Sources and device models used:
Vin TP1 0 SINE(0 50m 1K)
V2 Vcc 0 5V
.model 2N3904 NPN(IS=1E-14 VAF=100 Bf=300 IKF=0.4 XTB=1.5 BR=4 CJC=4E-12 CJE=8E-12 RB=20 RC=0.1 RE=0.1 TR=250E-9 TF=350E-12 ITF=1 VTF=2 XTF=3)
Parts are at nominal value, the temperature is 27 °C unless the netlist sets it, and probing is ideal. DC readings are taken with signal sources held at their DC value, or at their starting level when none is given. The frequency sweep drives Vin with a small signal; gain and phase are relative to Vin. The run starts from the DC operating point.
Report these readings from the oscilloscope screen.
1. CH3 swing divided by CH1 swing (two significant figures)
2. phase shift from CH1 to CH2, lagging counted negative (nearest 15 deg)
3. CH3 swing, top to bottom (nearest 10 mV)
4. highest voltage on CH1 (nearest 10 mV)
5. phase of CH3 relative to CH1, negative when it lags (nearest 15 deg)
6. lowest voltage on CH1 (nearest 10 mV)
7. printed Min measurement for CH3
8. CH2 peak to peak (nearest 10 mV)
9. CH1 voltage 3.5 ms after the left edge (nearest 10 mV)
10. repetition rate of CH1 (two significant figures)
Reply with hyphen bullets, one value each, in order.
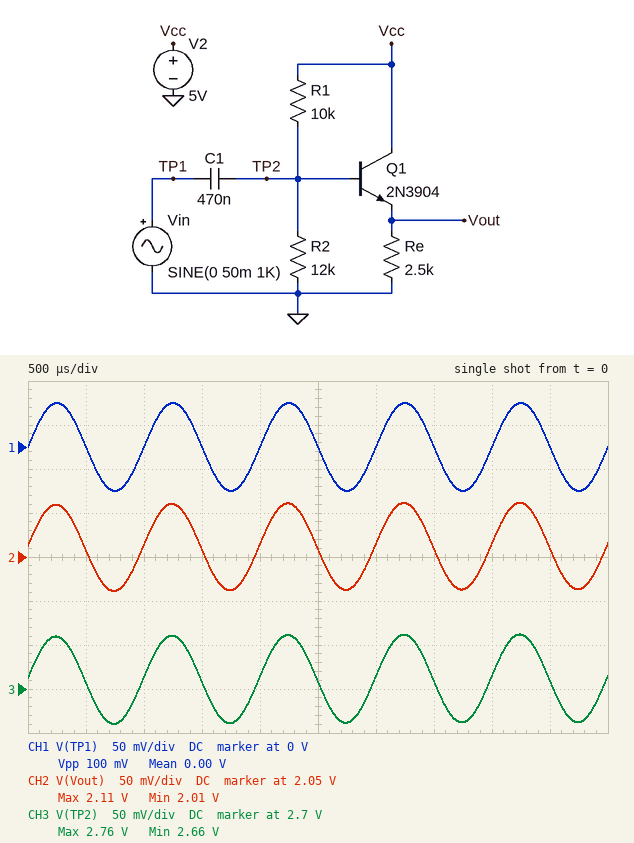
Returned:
- 1.0
- 0 deg
- 100 mV
- 50 mV
- 0 deg
- -50 mV
- 2.66 V
- 100 mV
- 0 V
- 1.0 kHz
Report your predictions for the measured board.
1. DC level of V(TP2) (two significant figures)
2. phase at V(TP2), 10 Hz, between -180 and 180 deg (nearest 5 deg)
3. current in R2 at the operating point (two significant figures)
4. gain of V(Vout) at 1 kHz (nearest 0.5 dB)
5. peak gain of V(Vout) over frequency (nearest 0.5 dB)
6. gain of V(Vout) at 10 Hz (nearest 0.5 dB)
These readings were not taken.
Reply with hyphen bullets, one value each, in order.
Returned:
- 2.7 V
- 80 deg
- 230 µA
- 0 dB
- 0 dB
- -16.0 dB
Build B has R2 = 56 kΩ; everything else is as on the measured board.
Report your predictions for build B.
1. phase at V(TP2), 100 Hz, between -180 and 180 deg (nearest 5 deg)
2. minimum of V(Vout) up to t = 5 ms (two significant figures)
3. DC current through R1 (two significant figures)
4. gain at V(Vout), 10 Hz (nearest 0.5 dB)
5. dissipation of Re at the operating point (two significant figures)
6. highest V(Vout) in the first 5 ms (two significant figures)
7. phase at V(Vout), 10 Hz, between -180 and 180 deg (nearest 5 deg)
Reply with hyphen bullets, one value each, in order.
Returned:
- 20 deg
- 3.5 V
- 80 µA
- -12.5 dB
- 5.0 mW
- 3.6 V
- 75 deg
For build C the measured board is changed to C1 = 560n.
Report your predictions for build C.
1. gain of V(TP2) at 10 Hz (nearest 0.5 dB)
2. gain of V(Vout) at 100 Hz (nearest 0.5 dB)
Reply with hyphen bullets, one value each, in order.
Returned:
- -14.5 dB
- -1.0 dB
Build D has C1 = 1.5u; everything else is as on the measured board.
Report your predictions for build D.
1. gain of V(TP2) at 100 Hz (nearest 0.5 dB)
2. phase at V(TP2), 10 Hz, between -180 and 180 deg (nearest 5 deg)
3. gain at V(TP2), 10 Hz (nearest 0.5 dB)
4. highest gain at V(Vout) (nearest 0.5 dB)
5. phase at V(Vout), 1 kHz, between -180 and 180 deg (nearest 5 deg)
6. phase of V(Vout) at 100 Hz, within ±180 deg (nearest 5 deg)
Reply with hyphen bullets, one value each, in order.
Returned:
- 0 dB
- 65 deg
- -7.0 dB
- 0 dB
- 0 deg
- 10 deg
